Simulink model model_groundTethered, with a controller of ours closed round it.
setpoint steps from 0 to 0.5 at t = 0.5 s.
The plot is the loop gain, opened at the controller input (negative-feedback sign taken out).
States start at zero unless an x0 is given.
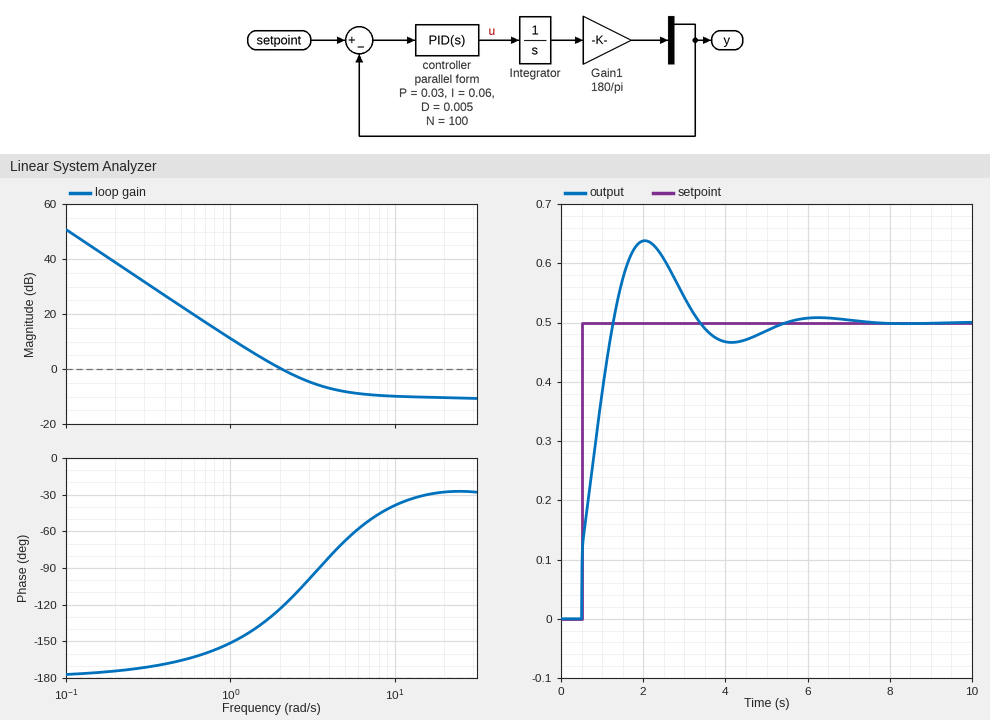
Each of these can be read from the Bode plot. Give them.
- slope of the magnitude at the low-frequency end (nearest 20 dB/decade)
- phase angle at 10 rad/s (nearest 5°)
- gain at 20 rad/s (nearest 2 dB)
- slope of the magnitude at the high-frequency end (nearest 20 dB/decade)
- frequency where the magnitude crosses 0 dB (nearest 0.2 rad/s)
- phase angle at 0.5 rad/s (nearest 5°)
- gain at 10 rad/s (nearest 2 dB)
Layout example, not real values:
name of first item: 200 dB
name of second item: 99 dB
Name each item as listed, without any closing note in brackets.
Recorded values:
slope of the magnitude at the low-frequency end: -40 dB/decade
phase angle at 10 rad/s: -40°
gain at 20 rad/s: -10 dB
slope of the magnitude at the high-frequency end: 0 dB/decade
frequency where the magnitude crosses 0 dB: 2.0 rad/s
phase angle at 0.5 rad/s: -165°
gain at 10 rad/s: -10 dB
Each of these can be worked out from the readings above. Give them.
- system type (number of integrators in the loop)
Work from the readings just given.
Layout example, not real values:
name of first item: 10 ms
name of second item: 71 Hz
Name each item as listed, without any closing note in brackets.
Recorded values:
system type: 2
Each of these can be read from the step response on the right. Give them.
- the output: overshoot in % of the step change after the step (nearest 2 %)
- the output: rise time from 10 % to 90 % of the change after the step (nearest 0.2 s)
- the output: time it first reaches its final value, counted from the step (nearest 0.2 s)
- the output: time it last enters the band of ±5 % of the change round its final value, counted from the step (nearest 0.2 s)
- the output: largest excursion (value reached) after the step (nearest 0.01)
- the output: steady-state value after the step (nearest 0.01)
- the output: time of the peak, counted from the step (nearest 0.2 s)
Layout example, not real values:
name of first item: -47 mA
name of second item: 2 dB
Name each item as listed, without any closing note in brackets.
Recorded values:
the output: overshoot in % of the step change after the step: 28 %
the output: rise time from 10 % to 90 % of the change after the step: 0.6 s
the output: time it first reaches its final value, counted from the step: 0.8 s
the output: time it last enters the band of ±5 % of the change round its final value, counted from the step: 4.2 s
the output: largest excursion (value reached) after the step: 0.64
the output: steady-state value after the step: 0.50
the output: time of the peak, counted from the step: 1.6 s
